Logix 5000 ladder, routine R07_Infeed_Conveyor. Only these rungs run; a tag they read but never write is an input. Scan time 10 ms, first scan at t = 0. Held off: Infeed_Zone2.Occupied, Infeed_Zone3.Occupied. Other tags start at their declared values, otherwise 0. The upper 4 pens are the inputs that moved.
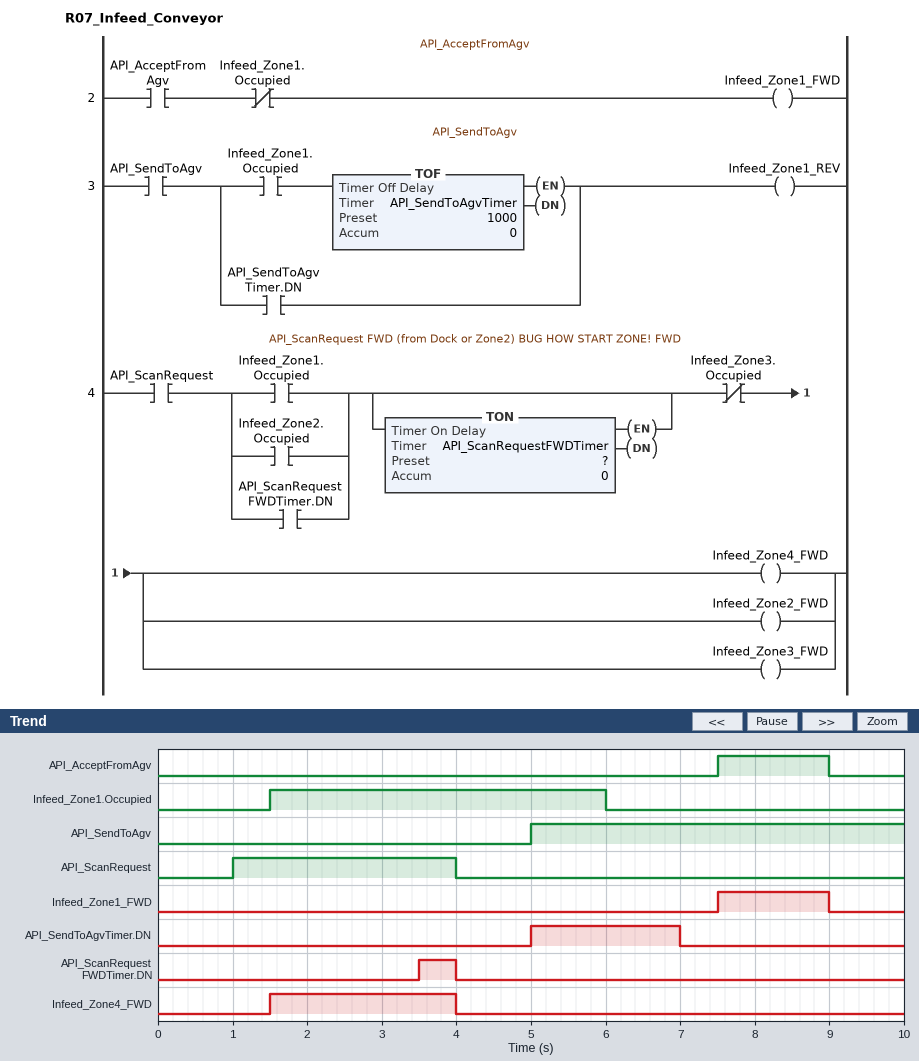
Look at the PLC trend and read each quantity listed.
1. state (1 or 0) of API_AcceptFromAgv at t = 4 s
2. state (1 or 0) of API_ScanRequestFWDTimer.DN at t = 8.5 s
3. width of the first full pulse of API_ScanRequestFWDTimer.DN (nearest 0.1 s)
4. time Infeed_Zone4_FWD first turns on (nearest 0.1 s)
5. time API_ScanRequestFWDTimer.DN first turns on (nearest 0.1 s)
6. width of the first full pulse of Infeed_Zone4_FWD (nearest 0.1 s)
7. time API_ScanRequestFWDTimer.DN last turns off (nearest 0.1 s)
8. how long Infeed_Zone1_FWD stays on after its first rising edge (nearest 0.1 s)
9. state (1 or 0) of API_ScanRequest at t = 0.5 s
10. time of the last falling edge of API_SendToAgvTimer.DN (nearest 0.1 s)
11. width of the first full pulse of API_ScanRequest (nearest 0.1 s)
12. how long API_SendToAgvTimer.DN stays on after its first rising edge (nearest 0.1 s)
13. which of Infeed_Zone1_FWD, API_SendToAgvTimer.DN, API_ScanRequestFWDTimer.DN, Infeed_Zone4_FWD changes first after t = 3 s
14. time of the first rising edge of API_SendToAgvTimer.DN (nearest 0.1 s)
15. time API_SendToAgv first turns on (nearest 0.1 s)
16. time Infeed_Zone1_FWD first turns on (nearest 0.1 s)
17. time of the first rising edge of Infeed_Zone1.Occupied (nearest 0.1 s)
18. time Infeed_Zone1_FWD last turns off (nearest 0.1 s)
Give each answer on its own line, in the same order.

0
0
0.5 s
1.5 s
3.5 s
2.5 s
4.0 s
1.5 s
0
7.0 s
3.0 s
2.0 s
API_ScanRequestFWDTimer.DN
5.0 s
5.0 s
7.5 s
1.5 s
9.0 s
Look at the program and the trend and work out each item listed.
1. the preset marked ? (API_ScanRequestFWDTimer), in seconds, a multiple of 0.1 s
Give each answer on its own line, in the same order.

2.0 s
